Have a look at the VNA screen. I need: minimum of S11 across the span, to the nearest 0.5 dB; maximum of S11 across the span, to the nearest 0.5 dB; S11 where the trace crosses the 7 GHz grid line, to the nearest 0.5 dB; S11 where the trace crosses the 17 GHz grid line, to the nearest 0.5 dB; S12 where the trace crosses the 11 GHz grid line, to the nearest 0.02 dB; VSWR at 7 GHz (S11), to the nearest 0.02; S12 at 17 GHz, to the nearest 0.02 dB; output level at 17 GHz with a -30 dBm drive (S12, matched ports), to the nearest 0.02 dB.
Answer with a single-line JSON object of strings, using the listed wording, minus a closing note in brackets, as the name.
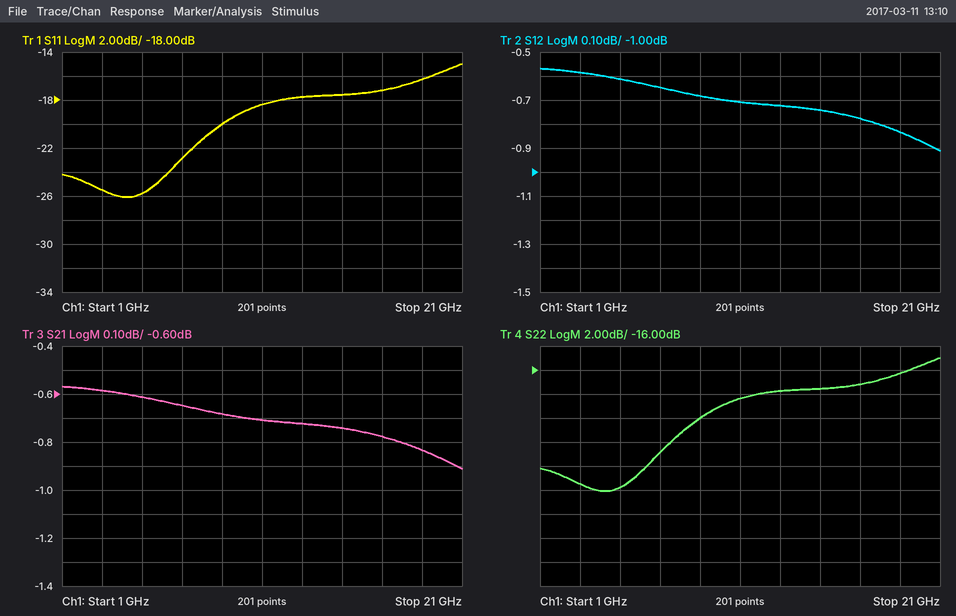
{"minimum of S11 across the span, to the nearest 0.5 dB": "-26.0 dB", "maximum of S11 across the span, to the nearest 0.5 dB": "-15.0 dB", "S11 where the trace crosses the 7 GHz grid line, to the nearest 0.5 dB": "-23.0 dB", "S11 where the trace crosses the 17 GHz grid line, to the nearest 0.5 dB": "-17.0 dB", "S12 where the trace crosses the 11 GHz grid line, to the nearest 0.02 dB": "-0.70 dB", "VSWR at 7 GHz (S11), to the nearest 0.02": "1.16", "S12 at 17 GHz, to the nearest 0.02 dB": "-0.78 dB", "output level at 17 GHz with a -30 dBm drive (S12, matched ports), to the nearest 0.02 dB": "-30.78 dBm"}
